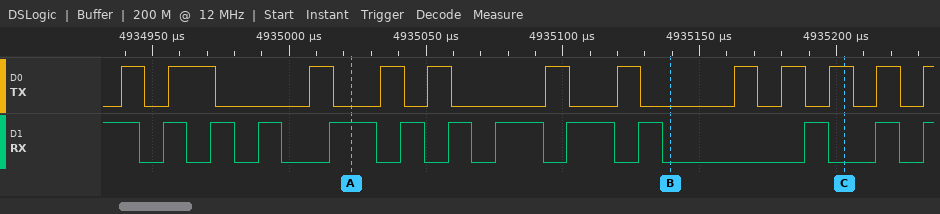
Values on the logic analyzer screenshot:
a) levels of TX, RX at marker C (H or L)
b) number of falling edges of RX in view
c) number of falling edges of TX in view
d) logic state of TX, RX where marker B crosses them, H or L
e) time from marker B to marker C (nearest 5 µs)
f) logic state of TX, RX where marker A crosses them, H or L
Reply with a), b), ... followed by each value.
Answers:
a) TX=H, RX=L
b) 12
c) 11
d) TX=L, RX=L
e) 65 µs
f) TX=L, RX=H
